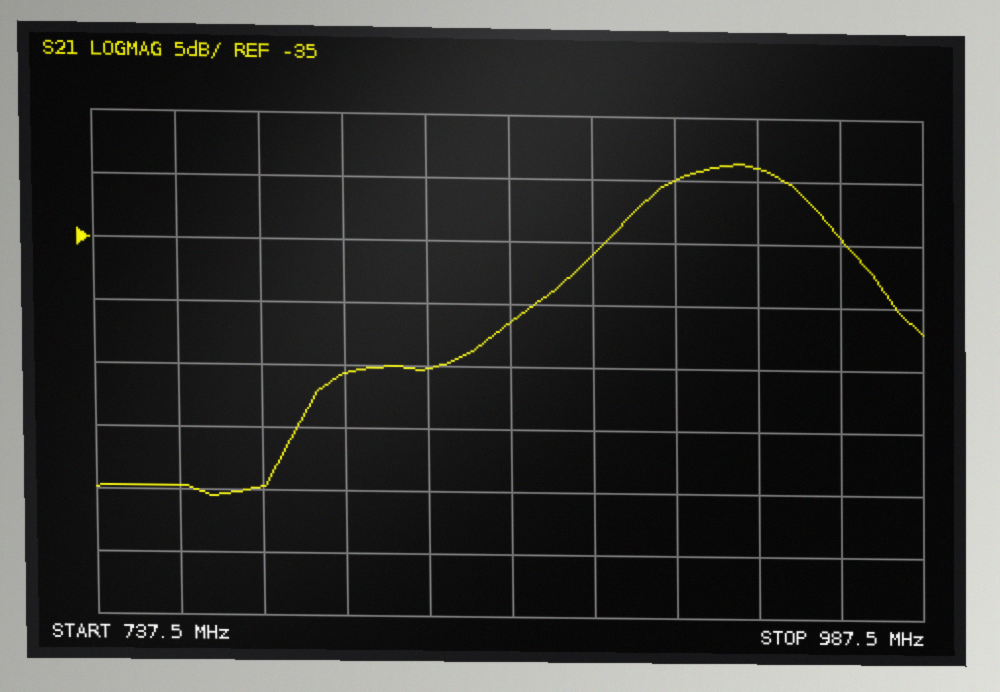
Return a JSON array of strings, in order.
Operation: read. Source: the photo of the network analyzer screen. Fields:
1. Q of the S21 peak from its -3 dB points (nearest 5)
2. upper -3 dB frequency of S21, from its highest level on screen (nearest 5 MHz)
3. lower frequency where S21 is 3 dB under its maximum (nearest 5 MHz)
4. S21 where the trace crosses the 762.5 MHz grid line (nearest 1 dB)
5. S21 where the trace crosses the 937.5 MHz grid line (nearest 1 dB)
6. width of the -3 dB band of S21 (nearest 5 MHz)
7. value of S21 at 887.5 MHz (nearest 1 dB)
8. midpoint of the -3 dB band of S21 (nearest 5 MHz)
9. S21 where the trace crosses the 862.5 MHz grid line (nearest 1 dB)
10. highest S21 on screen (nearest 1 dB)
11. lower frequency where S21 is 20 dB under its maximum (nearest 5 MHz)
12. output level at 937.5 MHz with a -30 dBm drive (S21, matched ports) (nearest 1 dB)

["20", "955 MHz", "905 MHz", "-55 dB", "-29 dB", "50 MHz", "-36 dB", "930 MHz", "-41 dB", "-29 dB", "800 MHz", "-59 dBm"]
